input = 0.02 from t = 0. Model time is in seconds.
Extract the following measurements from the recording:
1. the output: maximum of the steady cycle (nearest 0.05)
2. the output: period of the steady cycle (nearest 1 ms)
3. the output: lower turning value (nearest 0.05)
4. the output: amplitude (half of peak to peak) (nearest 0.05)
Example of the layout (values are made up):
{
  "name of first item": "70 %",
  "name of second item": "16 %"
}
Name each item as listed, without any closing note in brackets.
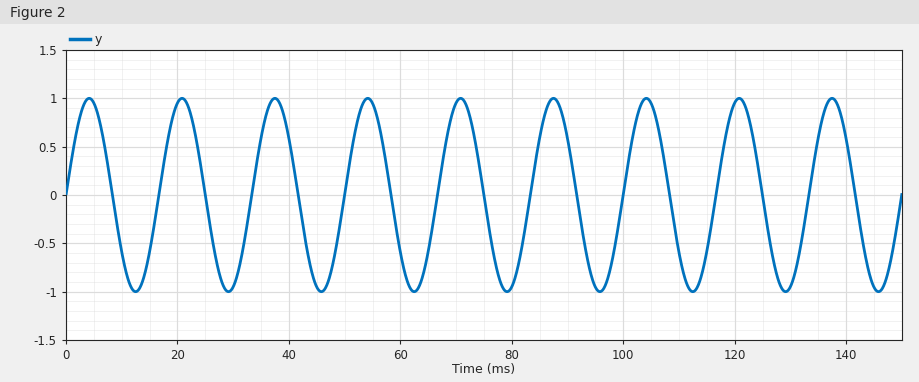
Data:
{
  "the output: maximum of the steady cycle": "1.00",
  "the output: period of the steady cycle": "17 ms",
  "the output: lower turning value": "-1.00",
  "the output: amplitude (half of peak to peak)": "1.00"
}
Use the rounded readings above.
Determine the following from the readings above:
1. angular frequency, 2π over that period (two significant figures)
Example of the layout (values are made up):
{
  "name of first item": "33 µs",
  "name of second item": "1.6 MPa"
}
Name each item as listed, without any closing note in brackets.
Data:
{
  "angular frequency, 2π over that period": "0.37 rad/ms"
}
